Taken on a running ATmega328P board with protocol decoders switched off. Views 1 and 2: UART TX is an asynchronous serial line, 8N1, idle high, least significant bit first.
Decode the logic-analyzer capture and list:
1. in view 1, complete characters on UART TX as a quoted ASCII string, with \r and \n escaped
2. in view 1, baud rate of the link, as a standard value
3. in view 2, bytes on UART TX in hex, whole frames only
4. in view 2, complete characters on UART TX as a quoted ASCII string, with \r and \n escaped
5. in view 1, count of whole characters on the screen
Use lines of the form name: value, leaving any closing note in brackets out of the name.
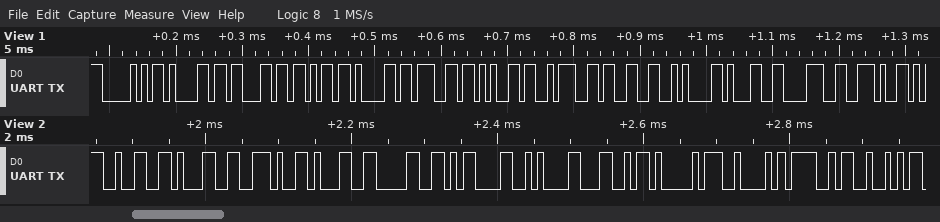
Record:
in view 1, complete characters on UART TX as a quoted ASCII string, with \r and \n escaped: "Package:3\n18."
in view 1, baud rate of the link, as a standard value: 115200 baud
in view 2, bytes on UART TX in hex, whole frames only: 0x32 0x31 0x2E 0x31 0x30 0x0D 0x0A 0x4C 0x41 0x42 0x4F 0x52
in view 2, complete characters on UART TX as a quoted ASCII string, with \r and \n escaped: "21.10\r\nLABOR"
in view 1, count of whole characters on the screen: 13
